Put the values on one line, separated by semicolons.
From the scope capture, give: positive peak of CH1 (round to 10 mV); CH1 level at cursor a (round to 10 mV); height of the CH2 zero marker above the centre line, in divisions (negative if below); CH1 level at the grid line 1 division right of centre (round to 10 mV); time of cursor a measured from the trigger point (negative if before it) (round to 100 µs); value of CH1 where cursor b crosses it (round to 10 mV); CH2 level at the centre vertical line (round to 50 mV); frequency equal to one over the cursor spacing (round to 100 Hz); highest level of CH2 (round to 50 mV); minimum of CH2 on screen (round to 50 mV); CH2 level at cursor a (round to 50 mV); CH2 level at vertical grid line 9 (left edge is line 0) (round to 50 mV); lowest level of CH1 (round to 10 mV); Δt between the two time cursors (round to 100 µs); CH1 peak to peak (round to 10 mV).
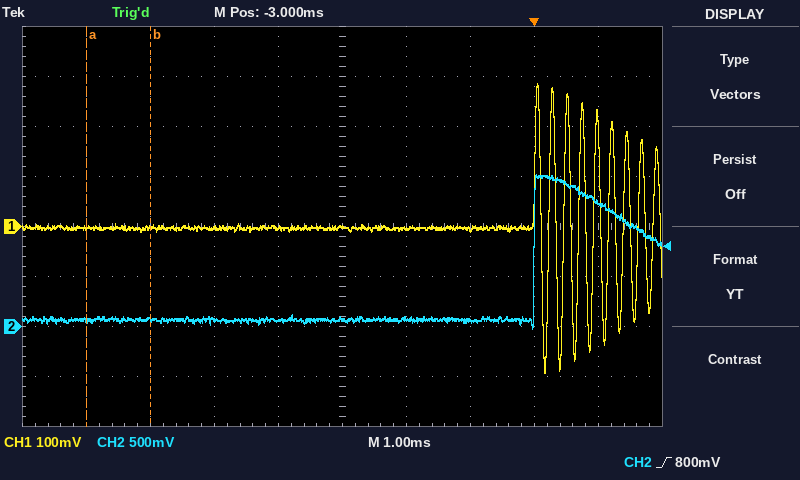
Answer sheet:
290 mV; 0 mV; -2.0 div; 0 mV; -7.0 ms; 0 mV; 100 mV; 1.0 kHz; 1.50 V; 0 mV; 50 mV; 1.25 V; -290 mV; 1.0 ms; 580 mV
